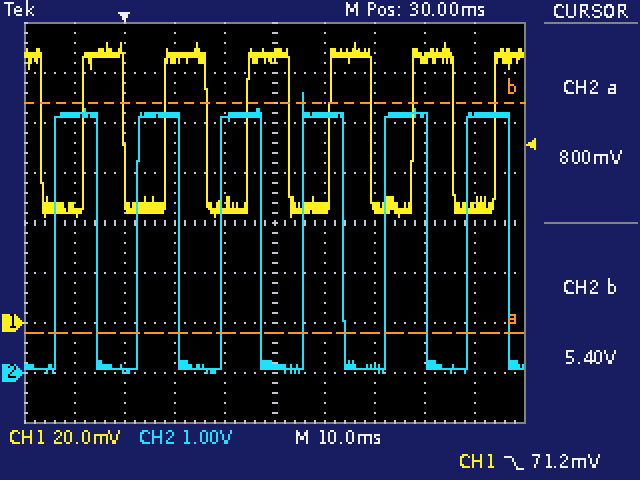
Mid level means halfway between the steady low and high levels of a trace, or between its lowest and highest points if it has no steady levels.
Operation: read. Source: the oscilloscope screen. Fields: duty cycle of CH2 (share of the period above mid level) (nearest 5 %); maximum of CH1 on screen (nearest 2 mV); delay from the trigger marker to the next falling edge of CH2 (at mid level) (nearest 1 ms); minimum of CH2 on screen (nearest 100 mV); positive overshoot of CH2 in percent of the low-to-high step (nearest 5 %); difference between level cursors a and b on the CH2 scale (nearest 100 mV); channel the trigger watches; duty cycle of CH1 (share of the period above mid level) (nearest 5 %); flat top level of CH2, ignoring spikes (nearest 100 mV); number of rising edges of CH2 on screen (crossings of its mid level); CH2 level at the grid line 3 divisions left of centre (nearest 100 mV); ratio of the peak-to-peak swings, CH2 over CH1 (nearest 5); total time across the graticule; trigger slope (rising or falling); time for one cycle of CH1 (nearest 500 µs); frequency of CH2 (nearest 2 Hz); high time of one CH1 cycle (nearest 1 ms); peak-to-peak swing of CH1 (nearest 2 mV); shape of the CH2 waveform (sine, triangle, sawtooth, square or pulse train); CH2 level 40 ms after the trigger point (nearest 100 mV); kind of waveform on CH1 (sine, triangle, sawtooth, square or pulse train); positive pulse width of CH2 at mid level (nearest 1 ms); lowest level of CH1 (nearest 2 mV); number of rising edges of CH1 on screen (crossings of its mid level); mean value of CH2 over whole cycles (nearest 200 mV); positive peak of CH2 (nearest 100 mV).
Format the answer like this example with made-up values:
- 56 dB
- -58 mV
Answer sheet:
- 50 %
- 112 mV
- 11 ms
- 0.0 V
- 10 %
- 4.6 V
- CH1
- 50 %
- 5.2 V
- 6
- 100 mV
- 80
- 100 ms
- falling
- 16.5 ms
- 60 Hz
- 8 ms
- 70 mV
- square
- 5.2 V
- square
- 8 ms
- 42 mV
- 6
- 2.6 V
- 5.6 V
